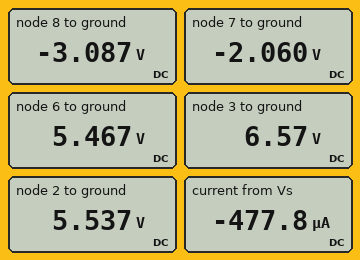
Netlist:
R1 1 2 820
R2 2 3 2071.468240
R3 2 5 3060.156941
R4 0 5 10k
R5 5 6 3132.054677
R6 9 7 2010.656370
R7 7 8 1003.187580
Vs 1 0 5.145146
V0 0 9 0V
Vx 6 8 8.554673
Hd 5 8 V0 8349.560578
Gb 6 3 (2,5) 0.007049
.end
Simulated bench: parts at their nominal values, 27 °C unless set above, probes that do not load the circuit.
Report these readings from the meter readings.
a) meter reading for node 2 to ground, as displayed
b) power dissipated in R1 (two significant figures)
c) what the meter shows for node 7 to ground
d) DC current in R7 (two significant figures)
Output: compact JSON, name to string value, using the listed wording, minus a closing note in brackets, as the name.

{"meter reading for node 2 to ground, as displayed": "5.537 V", "power dissipated in R1": "190 µW", "what the meter shows for node 7 to ground": "-2.060 V", "DC current in R7": "1.0 mA"}
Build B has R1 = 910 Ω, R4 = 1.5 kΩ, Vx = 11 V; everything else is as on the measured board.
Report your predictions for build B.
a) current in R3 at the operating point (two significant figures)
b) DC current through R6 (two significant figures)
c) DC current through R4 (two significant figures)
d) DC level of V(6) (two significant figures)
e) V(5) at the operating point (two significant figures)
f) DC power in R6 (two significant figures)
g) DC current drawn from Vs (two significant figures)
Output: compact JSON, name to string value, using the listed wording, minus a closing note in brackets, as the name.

{"current in R3 at the operating point": "88 µA", "DC current through R6": "710 µA", "DC current through R4": "2.5 mA", "DC level of V(6)": "8.9 V", "V(5) at the operating point": "3.8 V", "DC power in R6": "1.0 mW", "DC current drawn from Vs": "1.8 mA"}
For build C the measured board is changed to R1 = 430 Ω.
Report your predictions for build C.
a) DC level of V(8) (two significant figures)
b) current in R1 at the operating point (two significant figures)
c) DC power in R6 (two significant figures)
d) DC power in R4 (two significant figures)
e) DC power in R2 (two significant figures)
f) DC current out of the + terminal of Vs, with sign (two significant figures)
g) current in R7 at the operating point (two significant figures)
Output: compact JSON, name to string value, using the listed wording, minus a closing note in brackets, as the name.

{"DC level of V(8)": "-3.0 V", "current in R1 at the operating point": "460 µA", "DC power in R6": "2.0 mW", "DC power in R4": "2.8 mW", "DC power in R2": "480 µW", "DC current out of the + terminal of Vs, with sign": "-460 µA", "current in R7 at the operating point": "990 µA"}
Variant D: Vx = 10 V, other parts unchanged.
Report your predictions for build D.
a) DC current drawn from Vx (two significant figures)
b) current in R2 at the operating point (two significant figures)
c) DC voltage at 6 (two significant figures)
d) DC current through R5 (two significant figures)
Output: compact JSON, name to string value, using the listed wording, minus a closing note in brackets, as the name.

{"DC current drawn from Vx": "960 µA", "current in R2 at the operating point": "500 µA", "DC voltage at 6": "6.9 V", "DC current through R5": "460 µA"}
